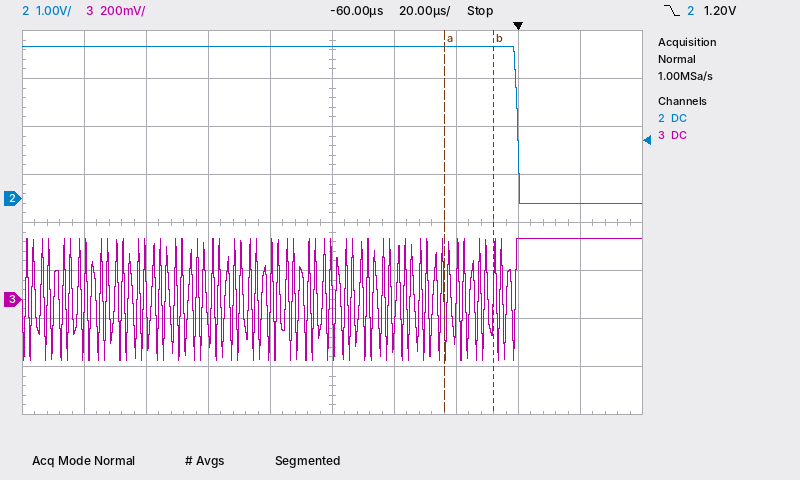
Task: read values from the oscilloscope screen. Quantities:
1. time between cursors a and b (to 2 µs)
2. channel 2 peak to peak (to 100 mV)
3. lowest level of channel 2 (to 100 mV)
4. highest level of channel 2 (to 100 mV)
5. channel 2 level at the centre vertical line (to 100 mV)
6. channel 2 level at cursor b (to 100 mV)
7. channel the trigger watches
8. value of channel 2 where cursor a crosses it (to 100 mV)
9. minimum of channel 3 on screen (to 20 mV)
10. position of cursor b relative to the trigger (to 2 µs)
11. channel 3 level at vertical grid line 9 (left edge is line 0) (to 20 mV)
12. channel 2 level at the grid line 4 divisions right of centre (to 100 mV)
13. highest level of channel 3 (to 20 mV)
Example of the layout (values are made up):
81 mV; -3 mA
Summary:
16 µs; 3.3 V; -100 mV; 3.2 V; 3.2 V; 3.2 V; channel 2; 3.2 V; -260 mV; -8 µs; 260 mV; -100 mV; 260 mV
